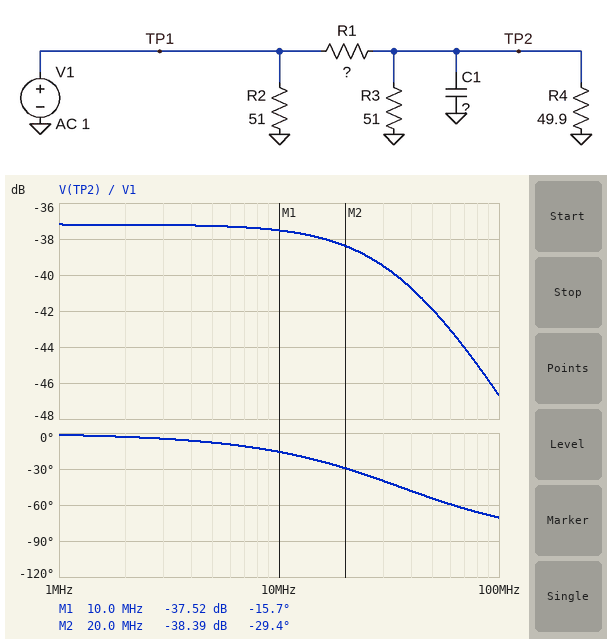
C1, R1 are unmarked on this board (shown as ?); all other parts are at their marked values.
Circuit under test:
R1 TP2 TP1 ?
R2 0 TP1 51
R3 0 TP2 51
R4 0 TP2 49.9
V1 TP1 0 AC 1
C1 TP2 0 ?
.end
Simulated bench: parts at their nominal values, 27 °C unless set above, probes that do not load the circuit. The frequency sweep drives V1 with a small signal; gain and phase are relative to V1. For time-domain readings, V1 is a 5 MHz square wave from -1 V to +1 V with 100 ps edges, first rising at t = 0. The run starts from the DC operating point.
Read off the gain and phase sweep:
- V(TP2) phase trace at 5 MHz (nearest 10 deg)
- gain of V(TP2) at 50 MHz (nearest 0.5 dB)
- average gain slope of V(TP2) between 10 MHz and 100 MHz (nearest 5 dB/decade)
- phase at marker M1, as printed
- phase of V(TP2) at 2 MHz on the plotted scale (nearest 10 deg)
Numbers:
-10 deg
-42.0 dB
-10 dB/decade
-15.7 deg
0 deg
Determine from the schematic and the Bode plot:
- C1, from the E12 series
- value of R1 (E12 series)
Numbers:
180 pF
1.8 kΩ
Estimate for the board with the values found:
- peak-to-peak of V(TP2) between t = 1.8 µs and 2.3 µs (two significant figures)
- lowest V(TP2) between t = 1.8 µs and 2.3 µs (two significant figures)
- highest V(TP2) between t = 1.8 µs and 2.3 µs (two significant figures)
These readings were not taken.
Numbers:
28 mV
-14 mV
14 mV
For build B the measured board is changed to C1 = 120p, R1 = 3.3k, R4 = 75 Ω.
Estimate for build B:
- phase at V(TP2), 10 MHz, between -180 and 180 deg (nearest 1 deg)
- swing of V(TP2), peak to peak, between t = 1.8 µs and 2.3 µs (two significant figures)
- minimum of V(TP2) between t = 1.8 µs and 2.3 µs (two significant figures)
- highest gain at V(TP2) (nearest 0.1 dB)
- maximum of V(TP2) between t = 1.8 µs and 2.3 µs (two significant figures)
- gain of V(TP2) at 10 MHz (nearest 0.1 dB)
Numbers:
-13 deg
18 mV
-9.1 mV
-40.8 dB
9.1 mV
-41.0 dB
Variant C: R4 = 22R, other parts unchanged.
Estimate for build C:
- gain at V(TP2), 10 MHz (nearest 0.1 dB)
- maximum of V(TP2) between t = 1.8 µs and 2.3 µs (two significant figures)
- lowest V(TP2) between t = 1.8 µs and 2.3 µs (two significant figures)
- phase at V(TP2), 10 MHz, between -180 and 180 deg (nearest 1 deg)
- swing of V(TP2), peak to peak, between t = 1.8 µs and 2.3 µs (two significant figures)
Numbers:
-41.6 dB
8.5 mV
-8.5 mV
-10 deg
17 mV
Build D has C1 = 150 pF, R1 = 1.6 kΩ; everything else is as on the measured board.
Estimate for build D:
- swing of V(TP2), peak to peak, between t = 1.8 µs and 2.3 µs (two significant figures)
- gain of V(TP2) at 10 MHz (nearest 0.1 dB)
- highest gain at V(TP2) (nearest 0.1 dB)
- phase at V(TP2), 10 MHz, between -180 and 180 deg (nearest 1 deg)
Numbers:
31 mV
-36.4 dB
-36.2 dB
-13 deg
